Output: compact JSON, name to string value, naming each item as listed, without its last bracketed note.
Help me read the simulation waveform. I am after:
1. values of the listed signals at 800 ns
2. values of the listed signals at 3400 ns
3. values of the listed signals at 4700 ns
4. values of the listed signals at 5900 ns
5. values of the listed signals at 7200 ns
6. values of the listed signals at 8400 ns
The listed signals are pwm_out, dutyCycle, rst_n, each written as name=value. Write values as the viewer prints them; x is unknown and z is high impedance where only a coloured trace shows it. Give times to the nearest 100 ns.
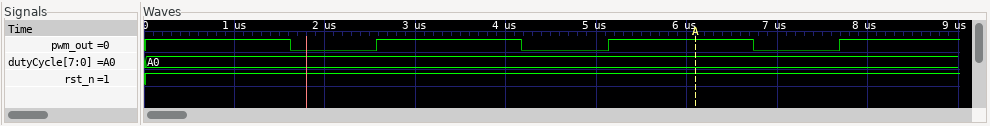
{"values of the listed signals at 800 ns": "pwm_out=1, dutyCycle=A0, rst_n=1", "values of the listed signals at 3400 ns": "pwm_out=1, dutyCycle=A0, rst_n=1", "values of the listed signals at 4700 ns": "pwm_out=0, dutyCycle=A0, rst_n=1", "values of the listed signals at 5900 ns": "pwm_out=1, dutyCycle=A0, rst_n=1", "values of the listed signals at 7200 ns": "pwm_out=0, dutyCycle=A0, rst_n=1", "values of the listed signals at 8400 ns": "pwm_out=1, dutyCycle=A0, rst_n=1"}
